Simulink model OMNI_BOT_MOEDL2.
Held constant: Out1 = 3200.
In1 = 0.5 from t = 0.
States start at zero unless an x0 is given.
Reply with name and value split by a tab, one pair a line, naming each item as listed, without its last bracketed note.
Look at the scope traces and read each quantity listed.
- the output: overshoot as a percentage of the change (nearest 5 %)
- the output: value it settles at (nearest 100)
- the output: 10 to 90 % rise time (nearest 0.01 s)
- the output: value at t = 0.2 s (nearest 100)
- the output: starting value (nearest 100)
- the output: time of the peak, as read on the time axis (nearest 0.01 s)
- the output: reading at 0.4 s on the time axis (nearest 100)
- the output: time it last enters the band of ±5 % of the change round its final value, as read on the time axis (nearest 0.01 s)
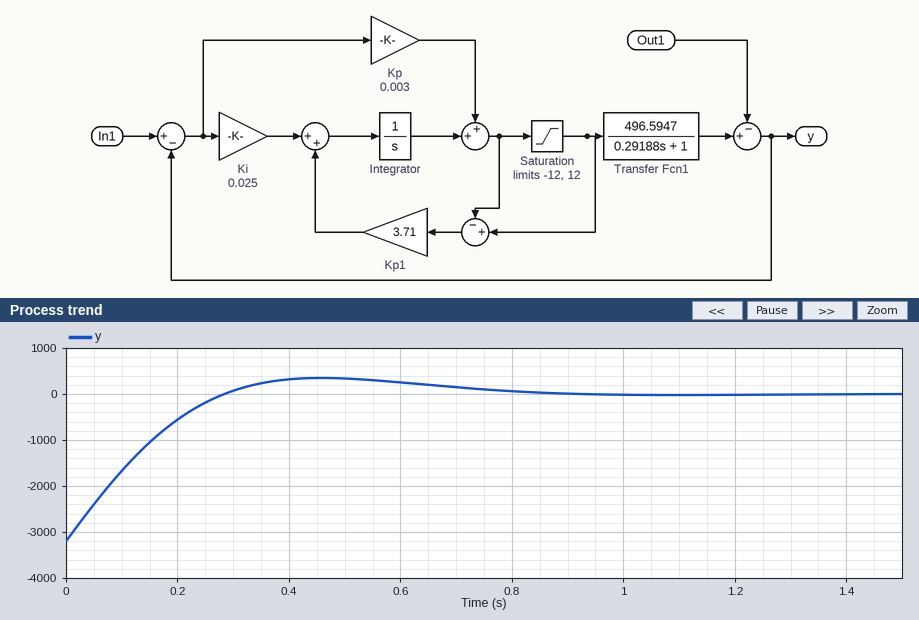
the output: overshoot as a percentage of the change	10 %
the output: value it settles at	0
the output: 10 to 90 % rise time	0.21 s
the output: value at t = 0.2 s	-600
the output: starting value	-3200
the output: time of the peak, as read on the time axis	0.46 s
the output: reading at 0.4 s on the time axis	300
the output: time it last enters the band of ±5 % of the change round its final value, as read on the time axis	0.69 s
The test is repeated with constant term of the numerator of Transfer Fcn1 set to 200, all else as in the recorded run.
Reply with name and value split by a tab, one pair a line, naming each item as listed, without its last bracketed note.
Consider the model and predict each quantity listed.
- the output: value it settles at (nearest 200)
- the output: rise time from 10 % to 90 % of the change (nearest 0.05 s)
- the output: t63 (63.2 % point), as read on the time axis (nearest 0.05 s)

the output: value it settles at	-800
the output: rise time from 10 % to 90 % of the change	0.65 s
the output: t63 (63.2 % point), as read on the time axis	0.30 s
